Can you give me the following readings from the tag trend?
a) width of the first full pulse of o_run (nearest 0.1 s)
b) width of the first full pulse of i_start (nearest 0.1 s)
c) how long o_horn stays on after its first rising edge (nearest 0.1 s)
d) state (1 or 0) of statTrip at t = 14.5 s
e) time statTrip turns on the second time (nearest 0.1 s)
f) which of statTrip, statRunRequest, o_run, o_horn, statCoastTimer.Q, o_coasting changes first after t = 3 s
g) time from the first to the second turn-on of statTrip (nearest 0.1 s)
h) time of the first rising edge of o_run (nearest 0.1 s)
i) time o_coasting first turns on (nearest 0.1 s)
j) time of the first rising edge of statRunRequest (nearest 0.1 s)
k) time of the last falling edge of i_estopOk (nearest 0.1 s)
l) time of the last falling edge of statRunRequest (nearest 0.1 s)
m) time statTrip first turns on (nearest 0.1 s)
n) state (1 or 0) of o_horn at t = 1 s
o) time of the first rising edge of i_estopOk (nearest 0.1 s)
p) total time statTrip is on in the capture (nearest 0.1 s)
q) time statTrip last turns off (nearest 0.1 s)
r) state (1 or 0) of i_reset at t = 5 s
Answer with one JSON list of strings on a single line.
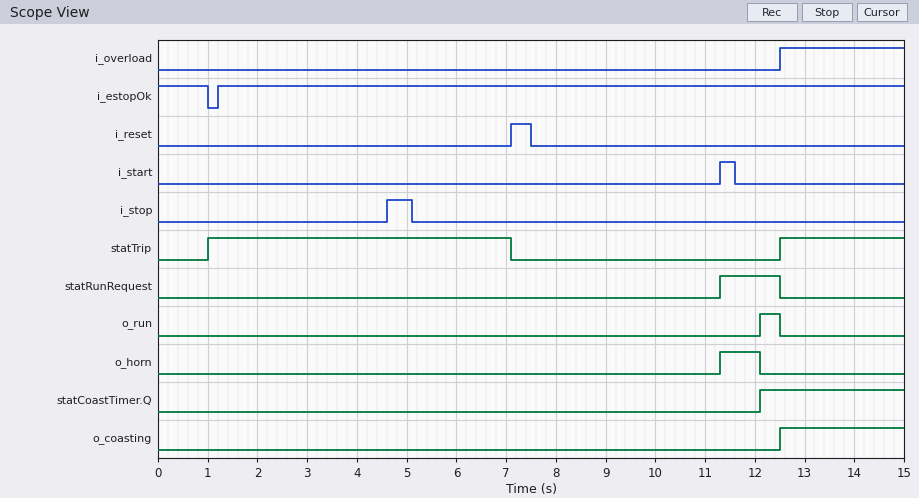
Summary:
["0.4 s", "0.3 s", "0.8 s", "1", "12.5 s", "statTrip", "11.5 s", "12.1 s", "12.5 s", "11.3 s", "1.0 s", "12.5 s", "1.0 s", "0", "1.2 s", "8.6 s", "7.1 s", "0"]
